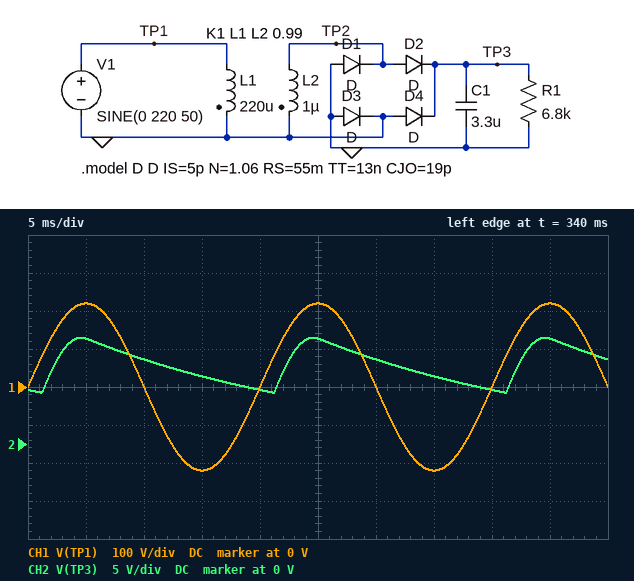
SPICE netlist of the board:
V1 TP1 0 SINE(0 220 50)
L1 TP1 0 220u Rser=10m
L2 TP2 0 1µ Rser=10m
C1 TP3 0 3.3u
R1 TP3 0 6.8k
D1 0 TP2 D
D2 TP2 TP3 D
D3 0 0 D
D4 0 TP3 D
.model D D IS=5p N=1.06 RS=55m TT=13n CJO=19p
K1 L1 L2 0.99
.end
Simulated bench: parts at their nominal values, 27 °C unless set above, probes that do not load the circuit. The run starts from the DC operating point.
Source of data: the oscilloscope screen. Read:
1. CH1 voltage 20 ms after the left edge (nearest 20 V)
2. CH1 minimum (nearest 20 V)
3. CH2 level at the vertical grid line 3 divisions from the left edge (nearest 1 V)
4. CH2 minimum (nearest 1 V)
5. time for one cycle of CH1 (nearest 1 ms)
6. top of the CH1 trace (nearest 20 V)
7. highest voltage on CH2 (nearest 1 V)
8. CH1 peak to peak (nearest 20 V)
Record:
0 V
-220 V
9 V
7 V
20 ms
220 V
14 V
440 V
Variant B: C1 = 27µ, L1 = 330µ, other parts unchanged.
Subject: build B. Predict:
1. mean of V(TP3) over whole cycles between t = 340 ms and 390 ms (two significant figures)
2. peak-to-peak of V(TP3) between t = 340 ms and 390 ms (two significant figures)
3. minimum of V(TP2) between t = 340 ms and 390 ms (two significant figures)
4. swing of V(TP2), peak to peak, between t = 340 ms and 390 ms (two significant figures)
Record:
11 V
1.1 V
-10 V
22 V
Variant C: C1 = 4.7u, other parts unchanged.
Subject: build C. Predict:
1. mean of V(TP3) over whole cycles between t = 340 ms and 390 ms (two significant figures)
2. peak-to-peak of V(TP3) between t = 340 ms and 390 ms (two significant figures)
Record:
11 V
5.7 V
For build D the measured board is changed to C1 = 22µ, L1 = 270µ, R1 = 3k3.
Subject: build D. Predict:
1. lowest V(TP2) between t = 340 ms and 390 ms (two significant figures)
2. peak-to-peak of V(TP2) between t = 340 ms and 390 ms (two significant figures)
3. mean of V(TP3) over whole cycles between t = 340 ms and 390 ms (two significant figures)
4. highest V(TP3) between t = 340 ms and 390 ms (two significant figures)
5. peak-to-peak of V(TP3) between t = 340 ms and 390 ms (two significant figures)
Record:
-11 V
24 V
11 V
13 V
2.7 V
